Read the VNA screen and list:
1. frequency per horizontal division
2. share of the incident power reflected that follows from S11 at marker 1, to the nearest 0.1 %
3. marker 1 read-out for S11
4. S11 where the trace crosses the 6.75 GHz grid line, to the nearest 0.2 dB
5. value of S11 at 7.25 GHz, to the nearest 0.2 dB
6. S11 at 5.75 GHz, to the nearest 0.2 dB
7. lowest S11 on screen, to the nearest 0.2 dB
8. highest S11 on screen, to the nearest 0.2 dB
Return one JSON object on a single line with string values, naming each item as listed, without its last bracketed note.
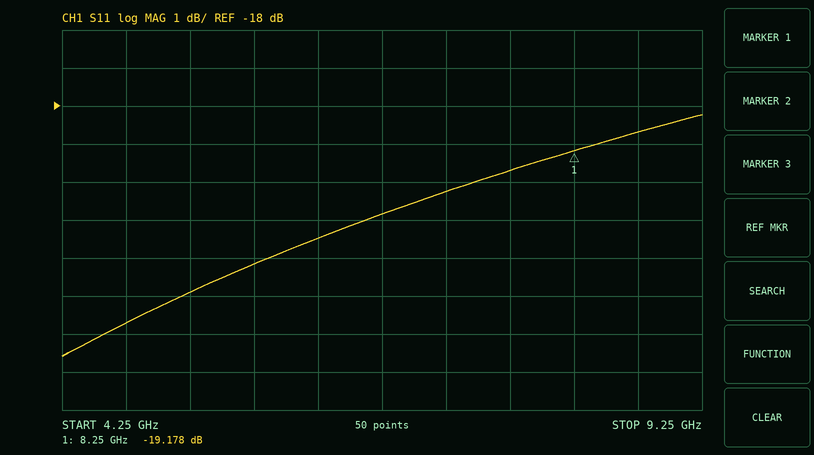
{"frequency per horizontal division": "500 MHz", "share of the incident power reflected that follows from S11 at marker 1, to the nearest 0.1 %": "1.2 %", "marker 1 read-out for S11": "-19.178 dB", "S11 where the trace crosses the 6.75 GHz grid line, to the nearest 0.2 dB": "-20.8 dB", "value of S11 at 7.25 GHz, to the nearest 0.2 dB": "-20.2 dB", "S11 at 5.75 GHz, to the nearest 0.2 dB": "-22.2 dB", "lowest S11 on screen, to the nearest 0.2 dB": "-24.6 dB", "highest S11 on screen, to the nearest 0.2 dB": "-18.2 dB"}
